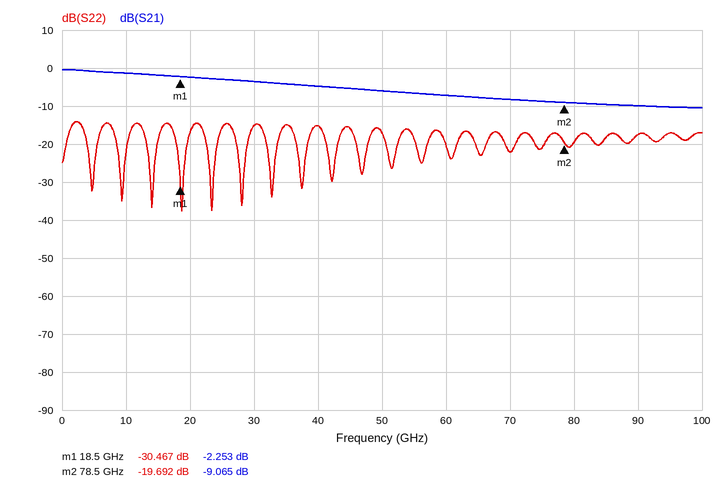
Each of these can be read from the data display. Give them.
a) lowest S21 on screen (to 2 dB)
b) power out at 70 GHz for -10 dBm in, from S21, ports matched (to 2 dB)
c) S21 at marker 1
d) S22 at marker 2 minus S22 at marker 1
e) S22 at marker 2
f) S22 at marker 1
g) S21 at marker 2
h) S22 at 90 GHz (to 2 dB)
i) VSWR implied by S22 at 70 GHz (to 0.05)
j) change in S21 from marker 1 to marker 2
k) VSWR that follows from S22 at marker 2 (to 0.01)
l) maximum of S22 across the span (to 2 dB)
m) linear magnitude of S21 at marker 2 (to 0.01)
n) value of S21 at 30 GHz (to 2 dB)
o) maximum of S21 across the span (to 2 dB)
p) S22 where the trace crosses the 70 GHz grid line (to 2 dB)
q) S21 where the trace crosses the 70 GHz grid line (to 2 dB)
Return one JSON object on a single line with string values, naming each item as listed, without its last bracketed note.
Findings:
{"lowest S21 on screen": "-10 dB", "power out at 70 GHz for -10 dBm in, from S21, ports matched": "-18 dBm", "S21 at marker 1": "-2.253 dB", "S22 at marker 2 minus S22 at marker 1": "10.775 dB", "S22 at marker 2": "-19.692 dB", "S22 at marker 1": "-30.467 dB", "S21 at marker 2": "-9.065 dB", "S22 at 90 GHz": "-18 dB", "VSWR implied by S22 at 70 GHz": "1.15", "change in S21 from marker 1 to marker 2": "-6.812 dB", "VSWR that follows from S22 at marker 2": "1.23", "maximum of S22 across the span": "-14 dB", "linear magnitude of S21 at marker 2": "0.35", "value of S21 at 30 GHz": "-4 dB", "maximum of S21 across the span": "0 dB", "S22 where the trace crosses the 70 GHz grid line": "-22 dB", "S21 where the trace crosses the 70 GHz grid line": "-8 dB"}
